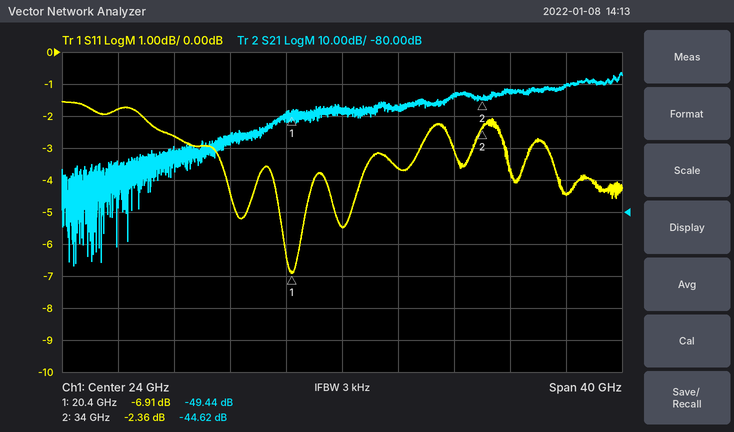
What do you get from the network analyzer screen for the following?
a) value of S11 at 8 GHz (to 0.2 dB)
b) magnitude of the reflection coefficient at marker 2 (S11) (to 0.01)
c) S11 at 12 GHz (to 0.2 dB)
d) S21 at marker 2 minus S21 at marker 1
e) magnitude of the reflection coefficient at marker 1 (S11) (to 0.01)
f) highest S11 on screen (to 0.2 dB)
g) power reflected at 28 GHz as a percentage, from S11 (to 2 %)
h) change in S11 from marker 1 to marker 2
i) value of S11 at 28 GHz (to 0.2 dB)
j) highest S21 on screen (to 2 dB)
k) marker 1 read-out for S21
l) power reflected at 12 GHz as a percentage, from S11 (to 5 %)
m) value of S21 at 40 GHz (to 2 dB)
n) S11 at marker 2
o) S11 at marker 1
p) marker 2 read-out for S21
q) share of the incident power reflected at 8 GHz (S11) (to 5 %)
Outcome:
-1.8 dB
0.76
-2.6 dB
4.82 dB
0.45
-1.6 dB
44 %
4.55 dB
-3.6 dB
-36 dB
-49.44 dB
55 %
-40 dB
-2.36 dB
-6.91 dB
-44.62 dB
65 %
